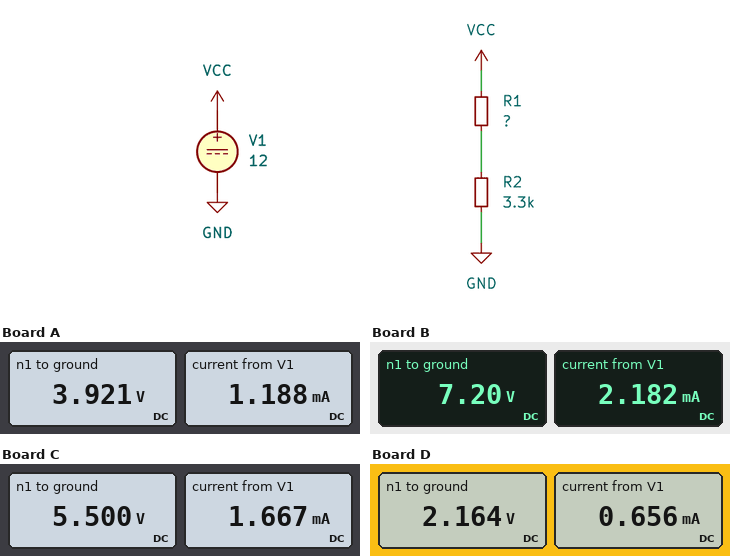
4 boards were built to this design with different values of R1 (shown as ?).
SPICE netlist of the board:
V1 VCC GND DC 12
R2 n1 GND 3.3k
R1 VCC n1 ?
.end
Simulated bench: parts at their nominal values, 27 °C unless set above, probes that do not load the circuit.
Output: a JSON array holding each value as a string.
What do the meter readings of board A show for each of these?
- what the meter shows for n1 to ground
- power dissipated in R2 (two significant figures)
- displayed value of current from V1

["3.921 V", "4.7 mW", "1.188 mA"]
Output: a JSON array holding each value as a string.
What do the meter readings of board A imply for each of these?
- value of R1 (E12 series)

["6.8 kΩ"]
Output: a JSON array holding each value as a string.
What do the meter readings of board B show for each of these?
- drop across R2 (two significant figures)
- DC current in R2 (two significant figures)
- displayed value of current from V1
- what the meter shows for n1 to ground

["7.2 V", "2.2 mA", "2.182 mA", "7.20 V"]
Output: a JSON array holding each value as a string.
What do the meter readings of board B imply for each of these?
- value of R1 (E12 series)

["2.2 kΩ"]
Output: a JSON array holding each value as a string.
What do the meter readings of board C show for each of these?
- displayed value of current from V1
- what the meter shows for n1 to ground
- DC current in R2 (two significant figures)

["1.667 mA", "5.500 V", "1.7 mA"]
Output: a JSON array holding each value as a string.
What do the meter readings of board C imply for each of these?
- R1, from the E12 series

["3.9 kΩ"]
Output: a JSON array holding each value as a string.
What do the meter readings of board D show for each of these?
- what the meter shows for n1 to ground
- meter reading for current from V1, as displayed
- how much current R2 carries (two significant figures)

["2.164 V", "0.656 mA", "660 µA"]
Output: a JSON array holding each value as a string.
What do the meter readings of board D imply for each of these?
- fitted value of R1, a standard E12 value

["15 kΩ"]
